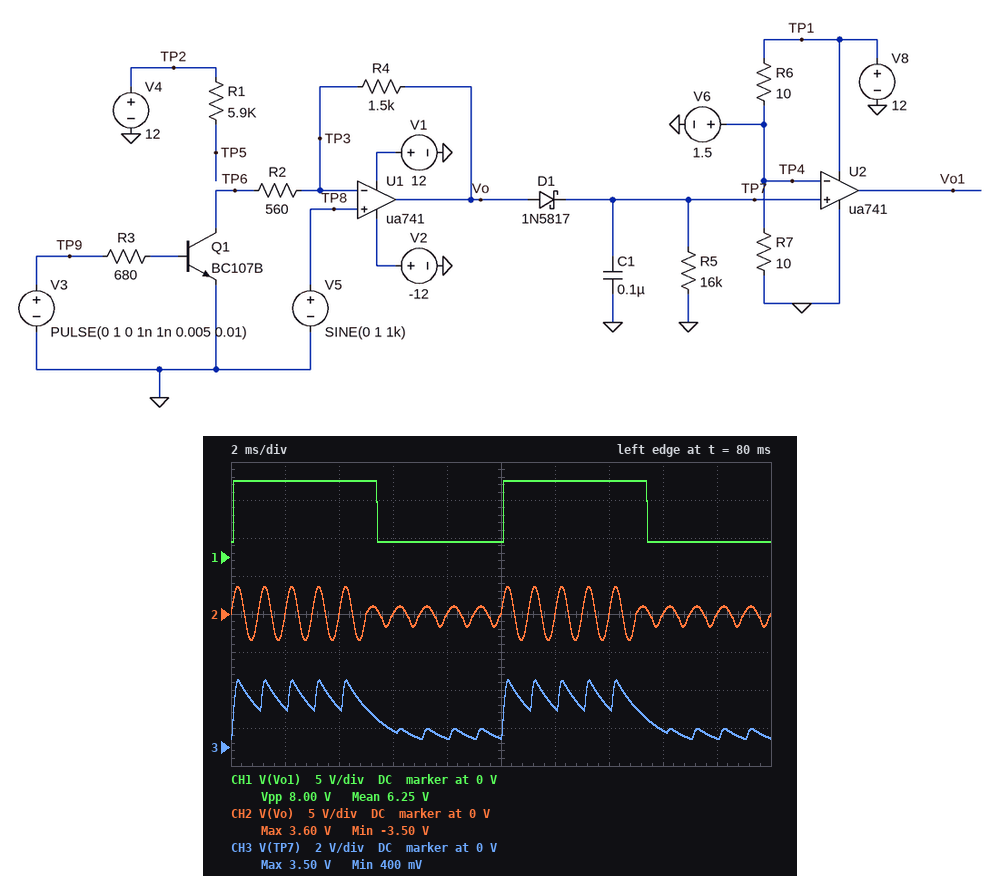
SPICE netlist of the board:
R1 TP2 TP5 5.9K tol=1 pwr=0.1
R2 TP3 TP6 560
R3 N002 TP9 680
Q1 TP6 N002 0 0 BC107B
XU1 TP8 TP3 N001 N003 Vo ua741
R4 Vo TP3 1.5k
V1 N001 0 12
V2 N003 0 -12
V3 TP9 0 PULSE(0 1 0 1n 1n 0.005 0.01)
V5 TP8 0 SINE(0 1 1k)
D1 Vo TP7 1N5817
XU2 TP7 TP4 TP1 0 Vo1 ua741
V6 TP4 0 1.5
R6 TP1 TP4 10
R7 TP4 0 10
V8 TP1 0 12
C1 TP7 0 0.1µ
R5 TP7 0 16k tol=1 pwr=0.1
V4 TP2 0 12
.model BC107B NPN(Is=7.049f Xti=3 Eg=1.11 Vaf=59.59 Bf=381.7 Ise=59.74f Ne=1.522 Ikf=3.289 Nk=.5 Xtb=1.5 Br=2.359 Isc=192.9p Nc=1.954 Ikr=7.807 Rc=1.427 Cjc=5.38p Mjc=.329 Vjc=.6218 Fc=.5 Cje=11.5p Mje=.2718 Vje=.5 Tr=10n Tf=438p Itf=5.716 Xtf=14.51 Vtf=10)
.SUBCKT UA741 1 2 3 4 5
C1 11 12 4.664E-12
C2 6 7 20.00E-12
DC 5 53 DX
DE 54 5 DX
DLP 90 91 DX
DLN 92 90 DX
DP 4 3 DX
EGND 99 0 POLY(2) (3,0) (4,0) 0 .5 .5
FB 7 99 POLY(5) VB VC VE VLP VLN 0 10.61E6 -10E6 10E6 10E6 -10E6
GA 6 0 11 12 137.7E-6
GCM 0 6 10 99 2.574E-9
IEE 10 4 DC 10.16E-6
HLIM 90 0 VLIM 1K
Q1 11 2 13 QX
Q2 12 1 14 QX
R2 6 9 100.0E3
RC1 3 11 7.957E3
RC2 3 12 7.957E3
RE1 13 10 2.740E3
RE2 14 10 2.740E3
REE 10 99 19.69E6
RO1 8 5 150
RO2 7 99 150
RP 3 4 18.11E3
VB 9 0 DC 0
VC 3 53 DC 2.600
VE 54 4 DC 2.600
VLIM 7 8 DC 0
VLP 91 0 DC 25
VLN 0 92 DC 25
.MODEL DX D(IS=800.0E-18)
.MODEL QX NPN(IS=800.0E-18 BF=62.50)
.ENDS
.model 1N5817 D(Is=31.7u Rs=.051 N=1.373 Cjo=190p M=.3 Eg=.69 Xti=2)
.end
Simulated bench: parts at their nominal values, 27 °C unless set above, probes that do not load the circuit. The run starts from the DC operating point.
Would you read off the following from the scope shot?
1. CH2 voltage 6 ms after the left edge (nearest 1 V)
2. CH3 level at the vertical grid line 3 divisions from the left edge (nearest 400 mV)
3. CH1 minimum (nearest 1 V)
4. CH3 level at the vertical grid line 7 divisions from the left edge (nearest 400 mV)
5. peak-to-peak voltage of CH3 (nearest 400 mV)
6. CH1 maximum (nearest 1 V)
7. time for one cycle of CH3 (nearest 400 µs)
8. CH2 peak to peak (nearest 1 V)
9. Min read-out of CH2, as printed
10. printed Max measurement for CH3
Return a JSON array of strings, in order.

["0 V", "800 mV", "2 V", "2.0 V", "3.2 V", "10 V", "10.0 ms", "7 V", "-3.50 V", "3.50 V"]
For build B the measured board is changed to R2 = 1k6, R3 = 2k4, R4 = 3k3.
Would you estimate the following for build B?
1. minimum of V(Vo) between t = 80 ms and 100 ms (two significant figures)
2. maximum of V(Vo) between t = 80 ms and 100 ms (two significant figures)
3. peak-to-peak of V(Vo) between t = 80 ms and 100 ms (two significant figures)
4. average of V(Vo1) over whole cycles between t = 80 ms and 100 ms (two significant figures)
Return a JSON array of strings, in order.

["-2.8 V", "3.0 V", "5.8 V", "6.0 V"]
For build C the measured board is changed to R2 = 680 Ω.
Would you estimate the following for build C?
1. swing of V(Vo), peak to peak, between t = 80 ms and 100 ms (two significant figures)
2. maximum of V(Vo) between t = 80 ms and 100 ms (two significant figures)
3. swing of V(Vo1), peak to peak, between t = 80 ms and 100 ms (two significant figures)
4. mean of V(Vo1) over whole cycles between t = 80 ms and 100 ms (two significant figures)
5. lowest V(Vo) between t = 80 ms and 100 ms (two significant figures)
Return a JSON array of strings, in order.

["6.2 V", "3.1 V", "8.0 V", "6.1 V", "-3.1 V"]
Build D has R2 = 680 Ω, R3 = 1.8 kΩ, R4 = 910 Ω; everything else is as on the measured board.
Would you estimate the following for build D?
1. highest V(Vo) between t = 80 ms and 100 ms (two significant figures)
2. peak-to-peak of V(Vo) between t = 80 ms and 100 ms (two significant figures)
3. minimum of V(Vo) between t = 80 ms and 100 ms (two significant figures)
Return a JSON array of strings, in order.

["2.3 V", "4.2 V", "-1.9 V"]
